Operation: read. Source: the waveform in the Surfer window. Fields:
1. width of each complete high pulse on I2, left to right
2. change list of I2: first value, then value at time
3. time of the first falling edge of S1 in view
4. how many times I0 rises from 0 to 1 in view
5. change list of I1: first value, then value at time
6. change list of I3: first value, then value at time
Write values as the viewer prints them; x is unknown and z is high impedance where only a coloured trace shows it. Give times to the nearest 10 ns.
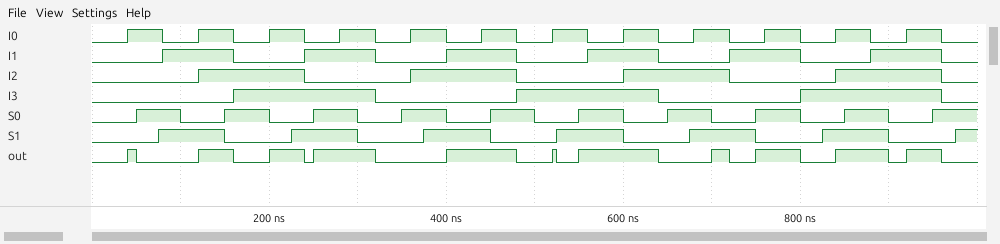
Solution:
120 ns, 120 ns, 120 ns, 120 ns
0, 1 at 120 ns, 0 at 240 ns, 1 at 360 ns, 0 at 480 ns, 1 at 600 ns, 0 at 720 ns, 1 at 840 ns, 0 at 960 ns
150 ns
12
0, 1 at 80 ns, 0 at 160 ns, 1 at 240 ns, 0 at 320 ns, 1 at 400 ns, 0 at 480 ns, 1 at 560 ns, 0 at 640 ns, 1 at 720 ns, 0 at 800 ns, 1 at 880 ns, 0 at 960 ns
0, 1 at 160 ns, 0 at 320 ns, 1 at 480 ns, 0 at 640 ns, 1 at 800 ns, 0 at 960 ns
